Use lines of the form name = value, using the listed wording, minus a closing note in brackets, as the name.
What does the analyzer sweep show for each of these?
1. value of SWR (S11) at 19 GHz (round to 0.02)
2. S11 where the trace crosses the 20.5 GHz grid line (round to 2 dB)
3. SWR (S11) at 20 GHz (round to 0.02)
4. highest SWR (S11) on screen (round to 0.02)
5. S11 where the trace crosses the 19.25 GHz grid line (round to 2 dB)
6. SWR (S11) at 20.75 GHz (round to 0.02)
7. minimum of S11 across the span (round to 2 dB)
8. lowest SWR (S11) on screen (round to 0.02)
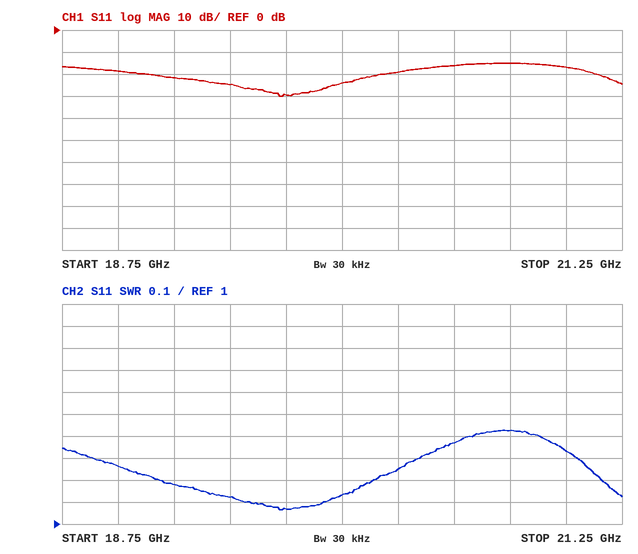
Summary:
value of SWR (S11) at 19 GHz = 1.26
S11 where the trace crosses the 20.5 GHz grid line = -16 dB
SWR (S11) at 20 GHz = 1.14
highest SWR (S11) on screen = 1.42
S11 where the trace crosses the 19.25 GHz grid line = -22 dB
SWR (S11) at 20.75 GHz = 1.42
minimum of S11 across the span = -30 dB
lowest SWR (S11) on screen = 1.06
